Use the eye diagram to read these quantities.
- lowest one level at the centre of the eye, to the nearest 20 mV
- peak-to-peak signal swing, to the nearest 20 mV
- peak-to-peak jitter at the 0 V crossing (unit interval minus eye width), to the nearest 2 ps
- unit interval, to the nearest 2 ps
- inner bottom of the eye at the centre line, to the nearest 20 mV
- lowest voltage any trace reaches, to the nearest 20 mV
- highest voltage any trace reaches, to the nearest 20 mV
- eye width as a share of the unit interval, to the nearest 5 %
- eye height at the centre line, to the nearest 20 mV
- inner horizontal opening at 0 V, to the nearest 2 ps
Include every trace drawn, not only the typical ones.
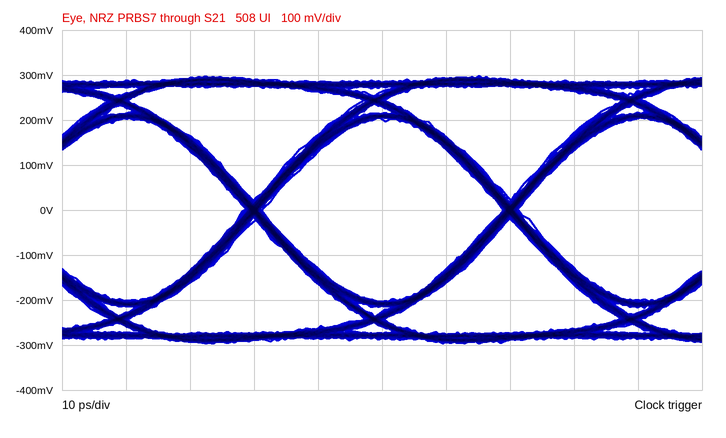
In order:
200 mV
600 mV
2 ps
40 ps
-200 mV
-300 mV
300 mV
95 %
400 mV
38 ps
